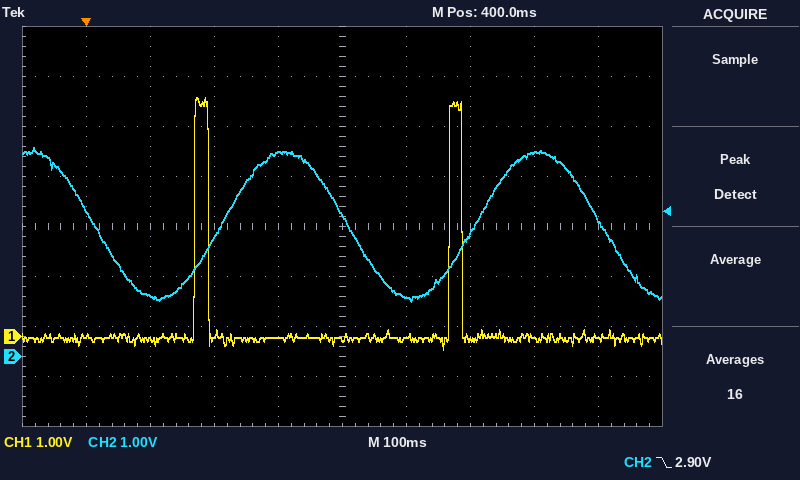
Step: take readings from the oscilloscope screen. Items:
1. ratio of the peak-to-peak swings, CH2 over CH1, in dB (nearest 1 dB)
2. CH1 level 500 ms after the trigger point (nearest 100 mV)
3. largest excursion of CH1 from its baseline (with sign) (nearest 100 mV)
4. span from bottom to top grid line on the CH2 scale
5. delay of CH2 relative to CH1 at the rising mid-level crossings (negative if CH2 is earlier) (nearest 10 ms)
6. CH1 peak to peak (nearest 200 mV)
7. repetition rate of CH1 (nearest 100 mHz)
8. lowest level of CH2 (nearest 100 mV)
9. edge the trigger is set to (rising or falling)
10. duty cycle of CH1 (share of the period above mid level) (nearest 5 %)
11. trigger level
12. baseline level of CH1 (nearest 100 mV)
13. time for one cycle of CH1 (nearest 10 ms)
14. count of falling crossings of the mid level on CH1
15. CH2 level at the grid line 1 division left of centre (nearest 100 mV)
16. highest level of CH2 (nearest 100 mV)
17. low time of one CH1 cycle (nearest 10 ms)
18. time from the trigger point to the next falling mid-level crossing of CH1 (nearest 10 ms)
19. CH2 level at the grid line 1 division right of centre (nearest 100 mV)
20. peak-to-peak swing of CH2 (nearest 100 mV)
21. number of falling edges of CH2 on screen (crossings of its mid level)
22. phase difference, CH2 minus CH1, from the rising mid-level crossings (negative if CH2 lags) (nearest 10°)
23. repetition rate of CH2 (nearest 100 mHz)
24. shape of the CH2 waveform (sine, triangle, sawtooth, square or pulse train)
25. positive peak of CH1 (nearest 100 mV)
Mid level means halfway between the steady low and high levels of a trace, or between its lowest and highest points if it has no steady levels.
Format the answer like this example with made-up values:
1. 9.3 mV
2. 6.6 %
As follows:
1. -4 dB
2. 0.0 V
3. +4.8 V
4. 8 V
5. +40 ms
6. 5.0 V
7. 2.5 Hz
8. 1.1 V
9. falling
10. 5 %
11. 2.90 V
12. 0.0 V
13. 400 ms
14. 2
15. 4.1 V
16. 4.2 V
17. 380 ms
18. 190 ms
19. 1.2 V
20. 3.1 V
21. 3
22. -40°
23. 2.5 Hz
24. sine
25. 4.8 V
